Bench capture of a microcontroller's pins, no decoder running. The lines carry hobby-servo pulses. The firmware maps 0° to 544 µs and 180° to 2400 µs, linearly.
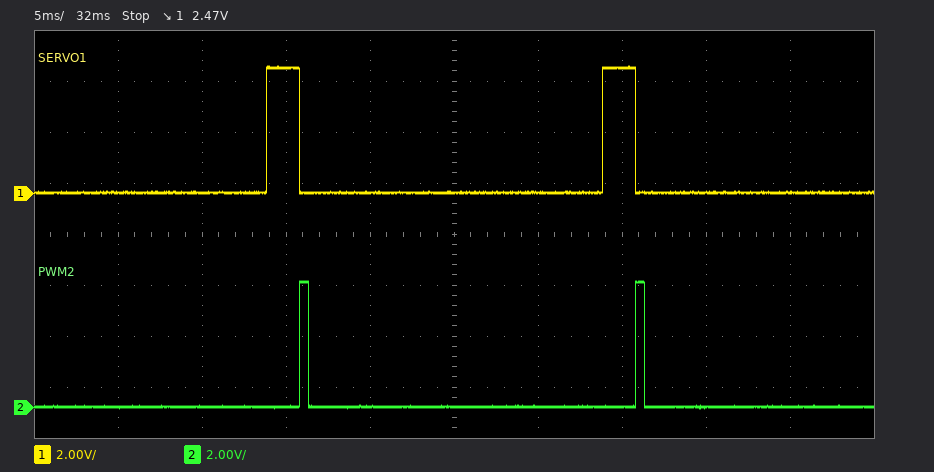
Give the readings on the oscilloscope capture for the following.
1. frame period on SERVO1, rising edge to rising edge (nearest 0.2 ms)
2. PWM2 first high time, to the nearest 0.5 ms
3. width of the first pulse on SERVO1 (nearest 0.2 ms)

20.0 ms
0.5 ms
2.0 ms
